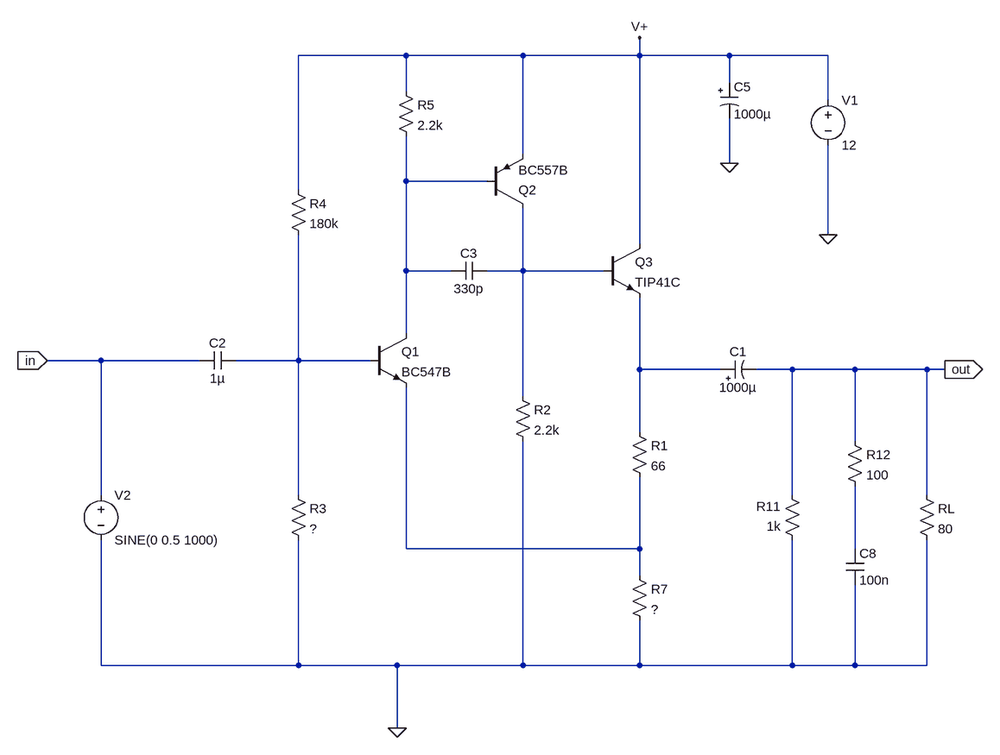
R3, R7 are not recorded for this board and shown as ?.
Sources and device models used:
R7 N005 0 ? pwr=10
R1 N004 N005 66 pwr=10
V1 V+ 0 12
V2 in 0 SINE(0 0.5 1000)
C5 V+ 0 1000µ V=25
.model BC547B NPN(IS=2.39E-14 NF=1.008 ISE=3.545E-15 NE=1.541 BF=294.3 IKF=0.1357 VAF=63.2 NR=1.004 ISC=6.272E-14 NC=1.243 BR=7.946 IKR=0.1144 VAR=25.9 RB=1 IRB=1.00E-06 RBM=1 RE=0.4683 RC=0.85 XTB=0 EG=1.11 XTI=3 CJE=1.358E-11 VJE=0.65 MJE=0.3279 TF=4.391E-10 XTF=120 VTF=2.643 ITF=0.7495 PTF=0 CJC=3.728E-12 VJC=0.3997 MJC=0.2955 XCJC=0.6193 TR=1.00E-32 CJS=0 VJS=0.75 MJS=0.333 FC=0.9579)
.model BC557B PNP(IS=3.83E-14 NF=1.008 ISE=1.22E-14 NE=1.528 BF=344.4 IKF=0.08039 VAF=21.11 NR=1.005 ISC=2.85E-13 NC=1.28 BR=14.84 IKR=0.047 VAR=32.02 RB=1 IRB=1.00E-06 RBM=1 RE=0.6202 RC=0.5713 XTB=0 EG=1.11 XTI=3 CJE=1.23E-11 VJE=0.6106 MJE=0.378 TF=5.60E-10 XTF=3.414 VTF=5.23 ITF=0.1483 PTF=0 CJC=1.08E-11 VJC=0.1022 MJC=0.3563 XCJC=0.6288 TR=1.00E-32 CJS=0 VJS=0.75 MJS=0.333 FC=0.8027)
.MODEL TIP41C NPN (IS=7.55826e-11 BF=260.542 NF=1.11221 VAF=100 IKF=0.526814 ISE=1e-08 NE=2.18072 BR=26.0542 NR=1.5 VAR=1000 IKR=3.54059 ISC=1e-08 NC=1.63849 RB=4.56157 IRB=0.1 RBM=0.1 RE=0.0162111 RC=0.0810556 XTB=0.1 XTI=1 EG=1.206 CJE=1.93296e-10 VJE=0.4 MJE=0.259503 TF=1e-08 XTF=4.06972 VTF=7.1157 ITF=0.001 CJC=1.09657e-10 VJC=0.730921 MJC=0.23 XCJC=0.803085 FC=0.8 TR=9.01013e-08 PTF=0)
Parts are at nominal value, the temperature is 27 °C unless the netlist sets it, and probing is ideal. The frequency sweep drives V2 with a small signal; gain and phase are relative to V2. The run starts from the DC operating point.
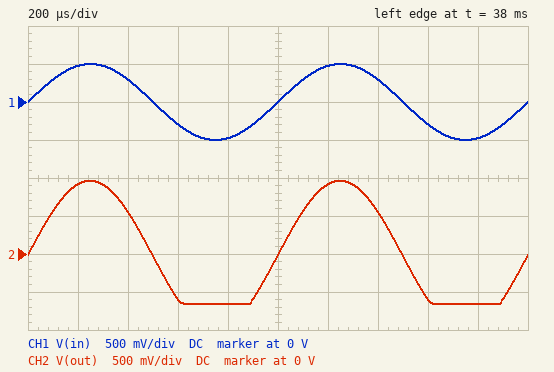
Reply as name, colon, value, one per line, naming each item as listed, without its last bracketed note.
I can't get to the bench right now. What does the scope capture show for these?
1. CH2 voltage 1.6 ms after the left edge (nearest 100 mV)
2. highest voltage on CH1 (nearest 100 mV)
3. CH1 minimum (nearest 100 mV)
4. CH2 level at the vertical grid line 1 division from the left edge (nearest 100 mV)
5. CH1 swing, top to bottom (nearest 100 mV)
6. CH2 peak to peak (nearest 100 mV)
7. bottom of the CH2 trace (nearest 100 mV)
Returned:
CH2 voltage 1.6 ms after the left edge: -600 mV
highest voltage on CH1: 500 mV
CH1 minimum: -500 mV
CH2 level at the vertical grid line 1 division from the left edge: 900 mV
CH1 swing, top to bottom: 1.0 V
CH2 peak to peak: 1.6 V
bottom of the CH2 trace: -700 mV
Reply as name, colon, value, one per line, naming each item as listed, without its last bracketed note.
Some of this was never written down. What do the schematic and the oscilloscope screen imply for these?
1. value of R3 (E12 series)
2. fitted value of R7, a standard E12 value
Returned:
value of R3: 27 kΩ
fitted value of R7, a standard E12 value: 68 Ω
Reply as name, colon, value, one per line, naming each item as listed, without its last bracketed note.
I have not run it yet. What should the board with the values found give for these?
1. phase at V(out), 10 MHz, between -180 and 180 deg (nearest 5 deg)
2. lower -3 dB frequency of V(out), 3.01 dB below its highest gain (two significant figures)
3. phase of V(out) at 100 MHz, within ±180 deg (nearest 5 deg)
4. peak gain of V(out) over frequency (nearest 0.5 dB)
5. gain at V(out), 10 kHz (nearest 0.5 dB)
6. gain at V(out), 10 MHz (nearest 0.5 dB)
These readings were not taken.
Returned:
phase at V(out), 10 MHz, between -180 and 180 deg: -125 deg
lower -3 dB frequency of V(out), 3.01 dB below its highest gain: 7.4 Hz
phase of V(out) at 100 MHz, within ±180 deg: 35 deg
peak gain of V(out) over frequency: 6.0 dB
gain at V(out), 10 kHz: 6.0 dB
gain at V(out), 10 MHz: -14.5 dB
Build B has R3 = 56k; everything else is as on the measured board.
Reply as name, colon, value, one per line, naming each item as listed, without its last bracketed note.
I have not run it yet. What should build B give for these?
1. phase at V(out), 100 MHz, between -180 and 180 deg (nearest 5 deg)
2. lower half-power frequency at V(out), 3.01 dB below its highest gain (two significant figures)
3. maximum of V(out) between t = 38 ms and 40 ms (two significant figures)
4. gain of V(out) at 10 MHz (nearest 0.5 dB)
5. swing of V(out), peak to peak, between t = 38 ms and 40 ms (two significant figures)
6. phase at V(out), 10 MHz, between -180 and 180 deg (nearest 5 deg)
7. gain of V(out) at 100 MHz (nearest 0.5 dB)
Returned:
phase at V(out), 100 MHz, between -180 and 180 deg: 40 deg
lower half-power frequency at V(out), 3.01 dB below its highest gain: 4.6 Hz
maximum of V(out) between t = 38 ms and 40 ms: 980 mV
gain of V(out) at 10 MHz: -12.5 dB
swing of V(out), peak to peak, between t = 38 ms and 40 ms: 2.0 V
phase at V(out), 10 MHz, between -180 and 180 deg: -105 deg
gain of V(out) at 100 MHz: -24.0 dB
